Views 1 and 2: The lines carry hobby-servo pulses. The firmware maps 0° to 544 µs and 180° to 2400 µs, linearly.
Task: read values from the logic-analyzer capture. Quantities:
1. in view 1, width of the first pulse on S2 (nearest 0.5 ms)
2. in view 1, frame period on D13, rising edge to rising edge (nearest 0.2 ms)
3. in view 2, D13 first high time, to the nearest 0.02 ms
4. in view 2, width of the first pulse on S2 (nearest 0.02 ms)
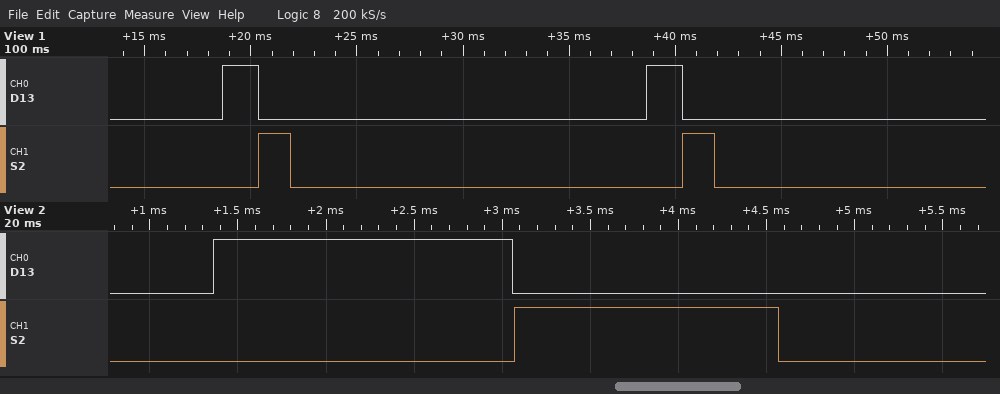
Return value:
1.5 ms
20.0 ms
1.70 ms
1.50 ms
